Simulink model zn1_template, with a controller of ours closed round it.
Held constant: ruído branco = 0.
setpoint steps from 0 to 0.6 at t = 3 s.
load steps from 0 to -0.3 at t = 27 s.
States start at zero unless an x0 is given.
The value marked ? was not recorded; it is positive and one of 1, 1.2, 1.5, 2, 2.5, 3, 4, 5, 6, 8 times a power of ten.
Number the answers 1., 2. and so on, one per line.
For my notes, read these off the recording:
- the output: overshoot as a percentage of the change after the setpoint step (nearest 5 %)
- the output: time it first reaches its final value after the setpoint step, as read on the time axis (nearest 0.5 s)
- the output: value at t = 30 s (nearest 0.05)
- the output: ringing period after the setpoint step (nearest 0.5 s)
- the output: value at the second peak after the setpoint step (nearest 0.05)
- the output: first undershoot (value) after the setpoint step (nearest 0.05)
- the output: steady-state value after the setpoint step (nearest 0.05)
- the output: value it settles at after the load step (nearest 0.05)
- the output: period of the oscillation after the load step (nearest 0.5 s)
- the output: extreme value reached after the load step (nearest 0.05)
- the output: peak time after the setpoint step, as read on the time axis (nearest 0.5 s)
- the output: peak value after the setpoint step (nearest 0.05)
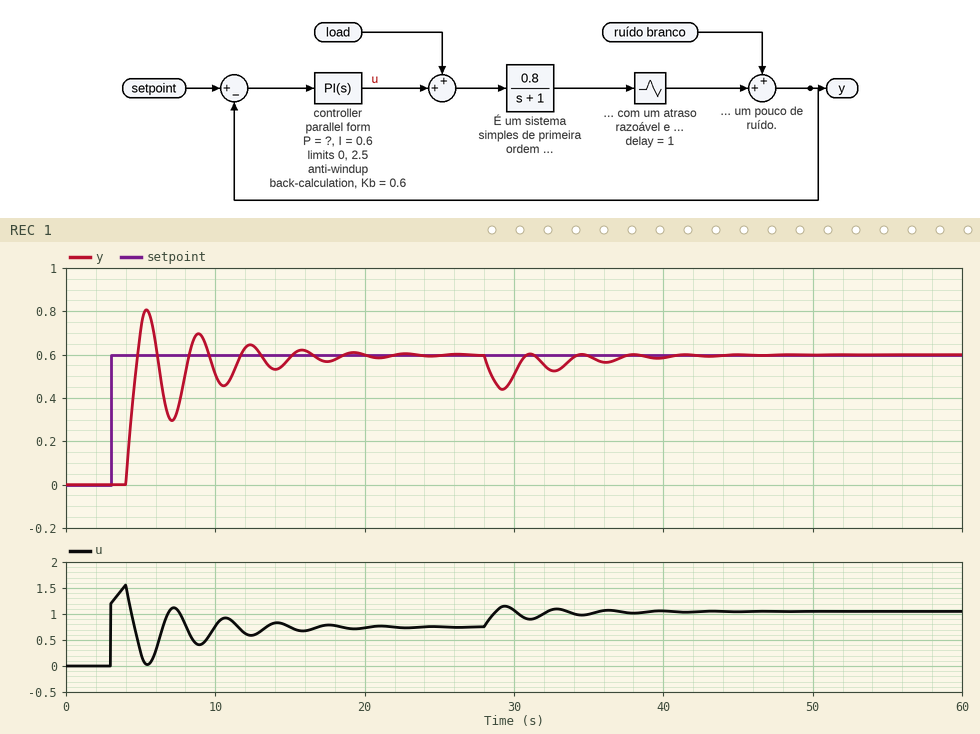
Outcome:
1. 35 %
2. 5.0 s
3. 0.50
4. 3.5 s
5. 0.70
6. 0.30
7. 0.60
8. 0.60
9. 3.5 s
10. 0.45
11. 5.5 s
12. 0.80
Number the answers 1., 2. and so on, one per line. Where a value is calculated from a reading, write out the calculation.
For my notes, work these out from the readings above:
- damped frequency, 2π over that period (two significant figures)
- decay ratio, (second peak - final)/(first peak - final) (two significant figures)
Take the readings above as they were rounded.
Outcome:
1. 2π / 3.5 = 1.8 rad/s
2. (0.7 - 0.6) / (0.8 - 0.6) = 0.50
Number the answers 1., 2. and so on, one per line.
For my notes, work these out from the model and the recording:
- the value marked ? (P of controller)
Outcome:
1. 2
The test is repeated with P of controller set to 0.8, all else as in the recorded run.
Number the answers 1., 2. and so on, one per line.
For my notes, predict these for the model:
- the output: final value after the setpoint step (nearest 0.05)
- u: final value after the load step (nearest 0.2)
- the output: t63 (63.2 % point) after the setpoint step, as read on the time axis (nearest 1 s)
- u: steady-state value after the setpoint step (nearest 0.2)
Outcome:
1. 0.60
2. 1.0
3. 5 s
4. 0.8
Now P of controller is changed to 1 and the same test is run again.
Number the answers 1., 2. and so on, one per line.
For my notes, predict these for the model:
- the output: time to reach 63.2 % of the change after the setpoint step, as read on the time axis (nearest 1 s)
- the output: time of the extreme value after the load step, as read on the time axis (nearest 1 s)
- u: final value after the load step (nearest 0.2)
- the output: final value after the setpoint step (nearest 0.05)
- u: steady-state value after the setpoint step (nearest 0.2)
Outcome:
1. 5 s
2. 29 s
3. 1.0
4. 0.60
5. 0.8
